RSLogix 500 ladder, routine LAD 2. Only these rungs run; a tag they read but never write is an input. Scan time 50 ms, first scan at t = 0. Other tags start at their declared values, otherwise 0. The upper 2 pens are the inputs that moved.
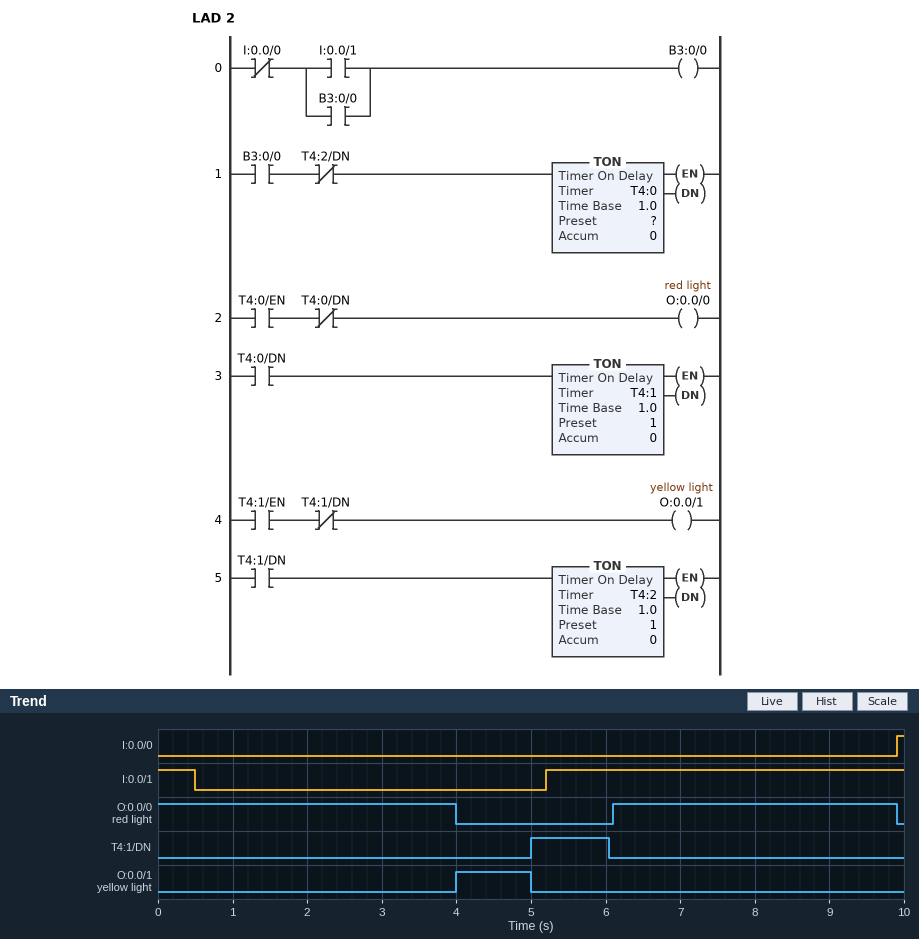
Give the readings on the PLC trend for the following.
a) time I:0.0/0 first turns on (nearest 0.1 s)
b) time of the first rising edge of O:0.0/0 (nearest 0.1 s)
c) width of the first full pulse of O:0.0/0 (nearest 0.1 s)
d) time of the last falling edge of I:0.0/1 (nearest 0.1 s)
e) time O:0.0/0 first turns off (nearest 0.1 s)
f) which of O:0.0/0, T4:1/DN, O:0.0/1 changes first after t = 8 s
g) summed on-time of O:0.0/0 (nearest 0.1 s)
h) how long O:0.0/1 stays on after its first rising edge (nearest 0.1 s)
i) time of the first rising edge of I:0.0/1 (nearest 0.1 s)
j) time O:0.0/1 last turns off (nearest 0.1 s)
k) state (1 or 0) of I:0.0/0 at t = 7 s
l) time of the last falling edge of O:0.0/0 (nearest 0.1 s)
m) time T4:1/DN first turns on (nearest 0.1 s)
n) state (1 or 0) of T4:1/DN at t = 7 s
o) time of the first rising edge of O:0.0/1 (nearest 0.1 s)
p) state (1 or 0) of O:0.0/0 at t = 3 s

9.9 s
6.1 s
3.8 s
0.5 s
4.0 s
O:0.0/0
7.8 s
1.0 s
5.2 s
5.0 s
0
9.9 s
5.0 s
0
4.0 s
1
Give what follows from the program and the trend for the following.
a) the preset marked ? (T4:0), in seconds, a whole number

4 s
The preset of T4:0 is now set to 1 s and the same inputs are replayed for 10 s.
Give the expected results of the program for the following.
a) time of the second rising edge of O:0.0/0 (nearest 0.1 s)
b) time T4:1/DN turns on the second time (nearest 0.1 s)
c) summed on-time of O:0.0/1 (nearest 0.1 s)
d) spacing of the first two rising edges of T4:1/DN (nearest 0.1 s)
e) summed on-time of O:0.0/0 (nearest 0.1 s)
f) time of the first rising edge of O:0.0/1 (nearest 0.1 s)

6.2 s
5.1 s
3.0 s
3.1 s
3.6 s
1.0 s
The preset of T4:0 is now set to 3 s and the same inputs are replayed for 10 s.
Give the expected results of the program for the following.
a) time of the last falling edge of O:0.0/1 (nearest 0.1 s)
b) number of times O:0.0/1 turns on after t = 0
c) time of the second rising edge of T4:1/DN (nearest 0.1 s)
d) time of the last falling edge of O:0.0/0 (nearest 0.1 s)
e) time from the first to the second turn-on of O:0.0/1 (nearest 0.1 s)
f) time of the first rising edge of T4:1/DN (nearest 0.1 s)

9.1 s
2
9.1 s
8.1 s
5.1 s
4.0 s
